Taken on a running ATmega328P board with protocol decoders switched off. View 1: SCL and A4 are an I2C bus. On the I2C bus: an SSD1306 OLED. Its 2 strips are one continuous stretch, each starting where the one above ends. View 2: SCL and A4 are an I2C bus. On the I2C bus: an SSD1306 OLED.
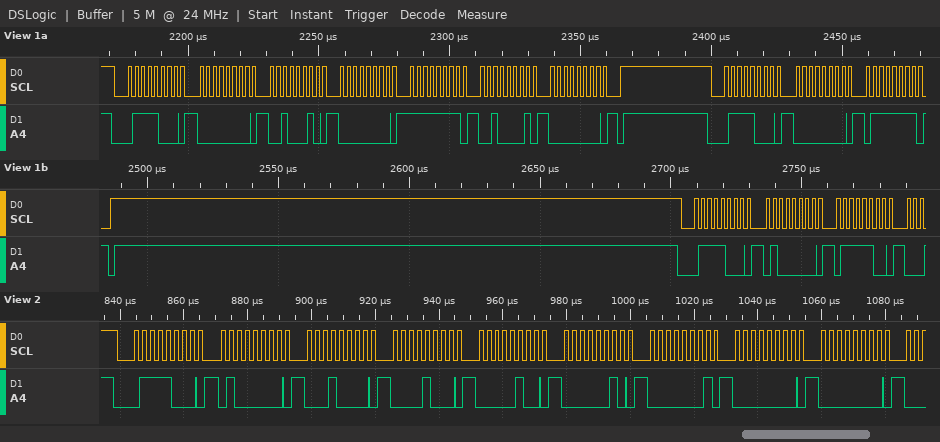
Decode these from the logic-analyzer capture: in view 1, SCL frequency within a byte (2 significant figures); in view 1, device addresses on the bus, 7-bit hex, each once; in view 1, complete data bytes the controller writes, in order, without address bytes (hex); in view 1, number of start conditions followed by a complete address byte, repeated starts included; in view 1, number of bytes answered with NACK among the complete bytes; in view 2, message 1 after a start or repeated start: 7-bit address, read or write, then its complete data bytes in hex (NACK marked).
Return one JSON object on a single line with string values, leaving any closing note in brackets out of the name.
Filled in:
{"in view 1, SCL frequency within a byte": "400 kHz", "in view 1, device addresses on the bus, 7-bit hex, each once": "0x3C", "in view 1, complete data bytes the controller writes, in order, without address bytes": "00 22 00 FF 21 00 00 7F 40 7C", "in view 1, number of start conditions followed by a complete address byte, repeated starts included": "3", "in view 1, number of bytes answered with NACK among the complete bytes": "0", "in view 2, message 1 after a start or repeated start: 7-bit address, read or write, then its complete data bytes in hex": "0x3C write: 40 10 08 04 02 01 00 00"}
